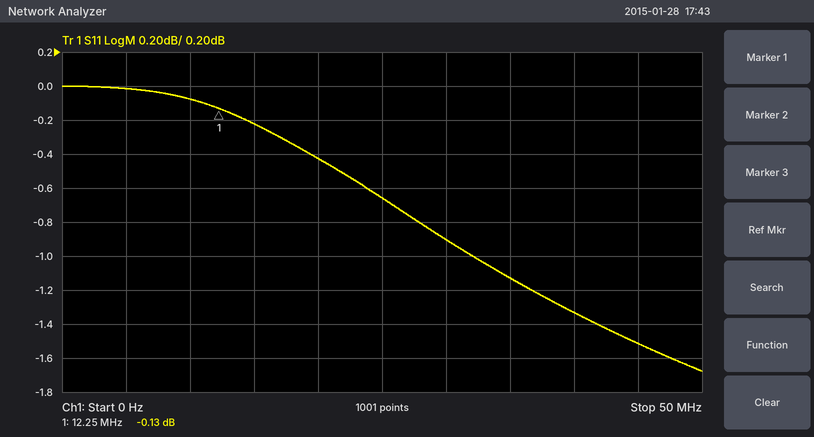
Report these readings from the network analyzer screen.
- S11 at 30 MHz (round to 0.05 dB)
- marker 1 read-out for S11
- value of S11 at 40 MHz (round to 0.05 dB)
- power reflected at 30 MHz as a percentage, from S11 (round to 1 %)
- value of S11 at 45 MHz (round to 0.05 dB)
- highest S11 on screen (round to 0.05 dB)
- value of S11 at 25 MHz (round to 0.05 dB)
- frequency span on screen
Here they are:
-0.90 dB
-0.13 dB
-1.35 dB
81 %
-1.50 dB
0.00 dB
-0.65 dB
50 MHz
